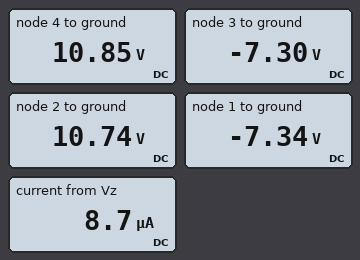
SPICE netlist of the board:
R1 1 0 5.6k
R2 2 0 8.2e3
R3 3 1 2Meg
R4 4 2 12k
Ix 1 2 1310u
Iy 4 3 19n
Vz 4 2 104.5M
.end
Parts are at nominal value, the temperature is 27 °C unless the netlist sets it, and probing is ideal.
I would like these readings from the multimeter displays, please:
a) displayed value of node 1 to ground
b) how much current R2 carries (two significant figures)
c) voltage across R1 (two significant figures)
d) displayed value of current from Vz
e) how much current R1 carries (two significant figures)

-7.34 V
1.3 mA
7.3 V
8.7 µA
1.3 mA
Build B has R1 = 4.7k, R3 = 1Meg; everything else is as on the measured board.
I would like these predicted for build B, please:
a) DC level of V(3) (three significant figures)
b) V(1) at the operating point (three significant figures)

-6.14 V
-6.16 V
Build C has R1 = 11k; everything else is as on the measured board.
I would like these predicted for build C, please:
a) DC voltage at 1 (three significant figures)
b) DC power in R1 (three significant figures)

-14.4 V
18.9 mW
